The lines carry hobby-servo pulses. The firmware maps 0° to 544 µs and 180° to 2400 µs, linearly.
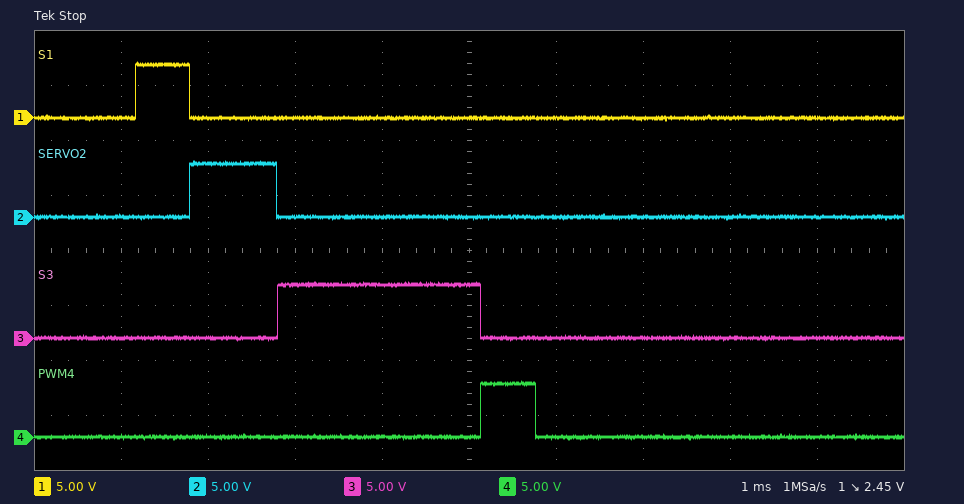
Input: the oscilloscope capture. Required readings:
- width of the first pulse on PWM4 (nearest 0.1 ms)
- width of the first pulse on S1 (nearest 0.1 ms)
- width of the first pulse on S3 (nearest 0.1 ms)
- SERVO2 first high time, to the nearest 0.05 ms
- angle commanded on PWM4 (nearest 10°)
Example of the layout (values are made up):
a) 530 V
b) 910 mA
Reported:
a) 0.6 ms
b) 0.6 ms
c) 2.3 ms
d) 1.00 ms
e) 10°
